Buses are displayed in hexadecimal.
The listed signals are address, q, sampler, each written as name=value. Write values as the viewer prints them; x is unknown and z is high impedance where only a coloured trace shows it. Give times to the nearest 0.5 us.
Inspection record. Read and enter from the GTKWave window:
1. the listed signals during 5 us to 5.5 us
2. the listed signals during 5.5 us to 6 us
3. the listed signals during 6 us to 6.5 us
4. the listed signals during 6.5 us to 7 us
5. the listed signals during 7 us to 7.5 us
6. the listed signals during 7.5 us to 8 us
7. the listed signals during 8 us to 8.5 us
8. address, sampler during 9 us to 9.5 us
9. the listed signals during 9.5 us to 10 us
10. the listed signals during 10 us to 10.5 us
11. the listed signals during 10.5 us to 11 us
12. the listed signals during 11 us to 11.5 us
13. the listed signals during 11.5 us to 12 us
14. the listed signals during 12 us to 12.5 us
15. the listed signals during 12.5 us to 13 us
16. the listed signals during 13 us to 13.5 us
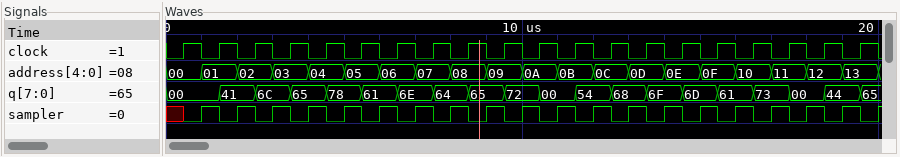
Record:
address=05, q=78, sampler=1
address=05, q=61, sampler=0
address=06, q=61, sampler=1
address=06, q=6E, sampler=0
address=07, q=6E, sampler=1
address=07, q=64, sampler=0
address=08, q=64, sampler=1
address=09, sampler=1
address=09, q=72, sampler=0
address=0A, q=72, sampler=1
address=0A, q=00, sampler=0
address=0B, q=00, sampler=1
address=0B, q=54, sampler=0
address=0C, q=54, sampler=1
address=0C, q=68, sampler=0
address=0D, q=68, sampler=1
